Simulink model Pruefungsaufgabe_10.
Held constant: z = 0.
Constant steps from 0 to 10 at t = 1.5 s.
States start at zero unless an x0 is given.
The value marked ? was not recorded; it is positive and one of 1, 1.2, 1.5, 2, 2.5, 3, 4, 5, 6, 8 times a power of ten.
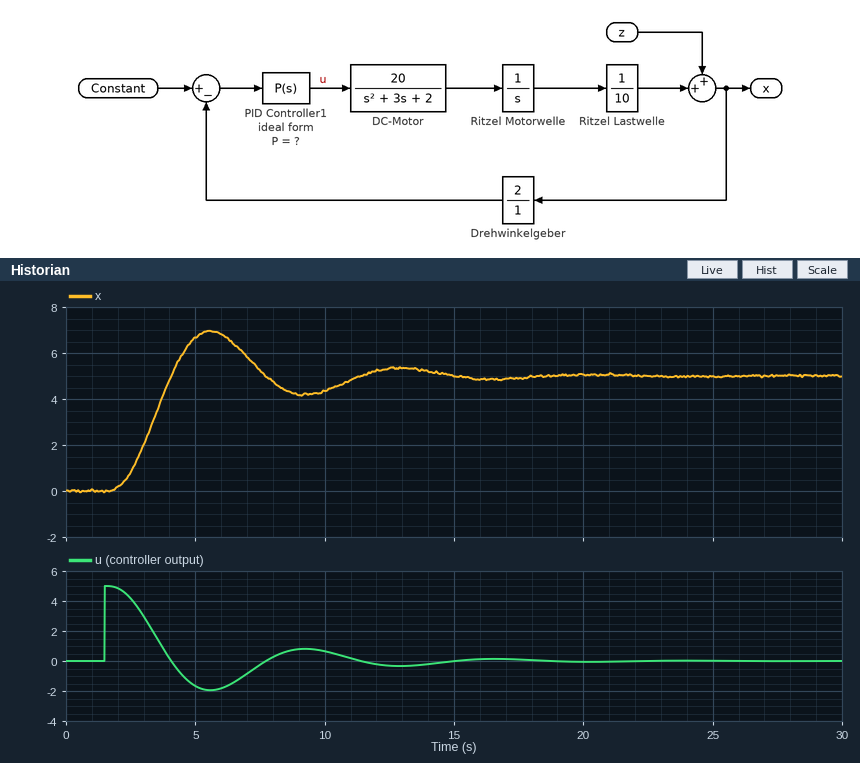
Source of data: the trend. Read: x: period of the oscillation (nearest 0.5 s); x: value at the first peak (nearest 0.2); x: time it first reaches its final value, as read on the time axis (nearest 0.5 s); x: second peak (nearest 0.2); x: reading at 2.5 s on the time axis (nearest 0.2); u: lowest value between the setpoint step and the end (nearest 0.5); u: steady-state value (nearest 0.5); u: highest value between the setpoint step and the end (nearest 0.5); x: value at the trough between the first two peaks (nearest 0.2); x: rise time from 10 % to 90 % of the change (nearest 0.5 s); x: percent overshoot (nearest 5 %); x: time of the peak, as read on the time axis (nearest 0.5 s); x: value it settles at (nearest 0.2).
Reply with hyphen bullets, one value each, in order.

- 7.5 s
- 7.0
- 4.0 s
- 5.4
- 0.8
- -2.0
- 0.0
- 5.0
- 4.2
- 1.5 s
- 40 %
- 5.5 s
- 5.0
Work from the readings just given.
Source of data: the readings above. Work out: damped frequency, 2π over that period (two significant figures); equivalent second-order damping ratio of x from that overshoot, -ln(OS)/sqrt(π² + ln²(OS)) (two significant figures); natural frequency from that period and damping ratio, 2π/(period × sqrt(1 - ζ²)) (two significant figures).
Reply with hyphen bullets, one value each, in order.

- 0.84 rad/s
- 0.28
- 0.87 rad/s
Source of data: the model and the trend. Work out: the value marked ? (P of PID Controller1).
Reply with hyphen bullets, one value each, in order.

- 0.5
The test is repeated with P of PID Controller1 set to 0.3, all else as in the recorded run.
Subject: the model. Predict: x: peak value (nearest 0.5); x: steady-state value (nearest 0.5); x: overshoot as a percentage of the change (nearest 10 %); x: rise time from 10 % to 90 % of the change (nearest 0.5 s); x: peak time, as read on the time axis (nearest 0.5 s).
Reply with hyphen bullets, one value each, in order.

- 6.0
- 5.0
- 20 %
- 2.5 s
- 7.0 s
